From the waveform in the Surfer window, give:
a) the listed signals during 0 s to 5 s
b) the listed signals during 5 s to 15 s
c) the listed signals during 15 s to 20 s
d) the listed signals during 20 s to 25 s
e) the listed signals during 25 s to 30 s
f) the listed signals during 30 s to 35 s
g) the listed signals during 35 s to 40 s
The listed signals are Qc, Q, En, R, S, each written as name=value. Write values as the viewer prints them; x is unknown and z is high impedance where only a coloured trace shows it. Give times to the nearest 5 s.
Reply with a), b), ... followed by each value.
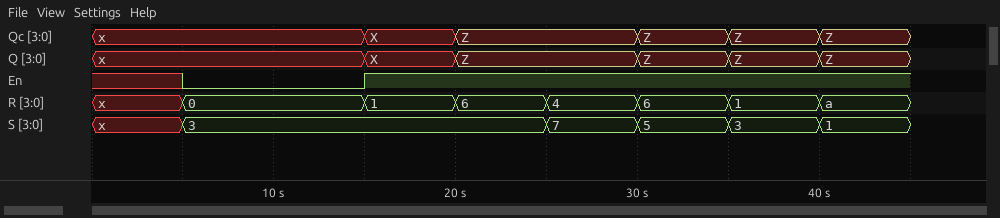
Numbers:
a) Qc=x, Q=x, En=x, R=x, S=x
b) Qc=x, Q=x, En=0, R=0, S=3
c) Qc=X, Q=X, En=1, R=1, S=3
d) Qc=Z, Q=Z, En=1, R=6, S=3
e) Qc=Z, Q=Z, En=1, R=4, S=7
f) Qc=Z, Q=Z, En=1, R=6, S=5
g) Qc=Z, Q=Z, En=1, R=1, S=3
